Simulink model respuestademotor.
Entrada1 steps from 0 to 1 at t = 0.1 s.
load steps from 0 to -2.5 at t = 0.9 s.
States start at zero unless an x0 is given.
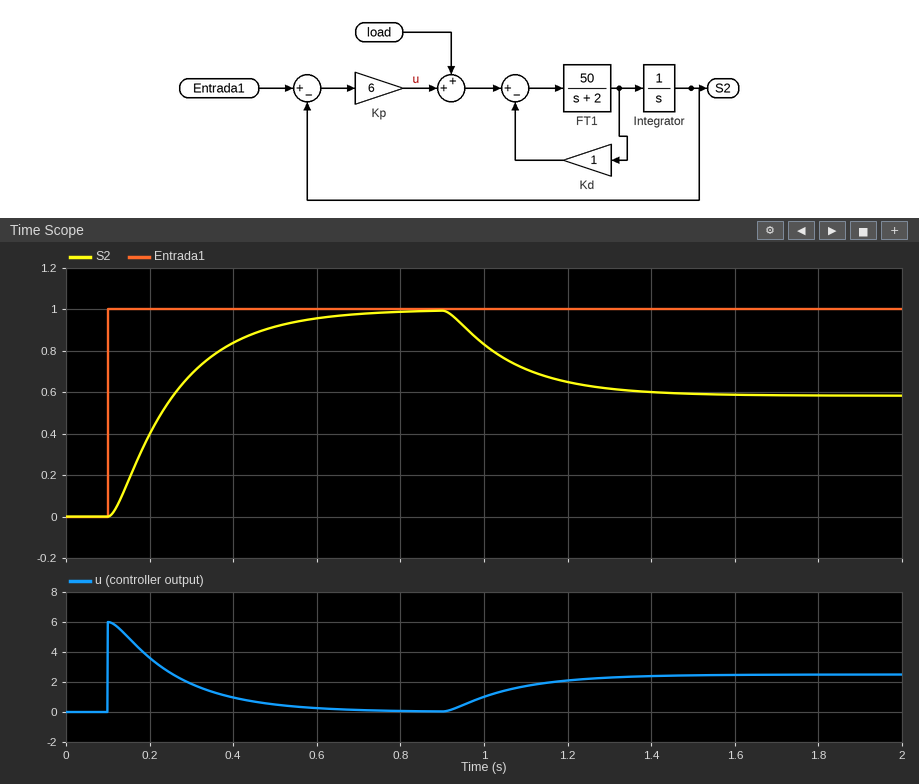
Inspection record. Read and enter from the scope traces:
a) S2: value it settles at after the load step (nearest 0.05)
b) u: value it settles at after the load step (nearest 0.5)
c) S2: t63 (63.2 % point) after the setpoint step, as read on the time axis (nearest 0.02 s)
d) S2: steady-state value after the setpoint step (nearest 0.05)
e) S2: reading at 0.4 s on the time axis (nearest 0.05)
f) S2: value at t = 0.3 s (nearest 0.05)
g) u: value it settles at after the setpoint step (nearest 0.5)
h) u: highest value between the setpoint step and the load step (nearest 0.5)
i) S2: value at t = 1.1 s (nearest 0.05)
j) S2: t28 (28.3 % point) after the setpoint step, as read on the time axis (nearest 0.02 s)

0.60
2.5
0.28 s
1.00
0.85
0.70
0.0
6.0
0.70
0.18 s
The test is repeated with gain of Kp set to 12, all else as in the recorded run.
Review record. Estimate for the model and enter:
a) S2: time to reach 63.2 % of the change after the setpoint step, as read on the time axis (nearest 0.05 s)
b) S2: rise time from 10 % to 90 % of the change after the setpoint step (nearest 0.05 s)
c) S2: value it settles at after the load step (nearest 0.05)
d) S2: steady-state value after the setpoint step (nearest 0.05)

0.20 s
0.15 s
0.80
1.00
